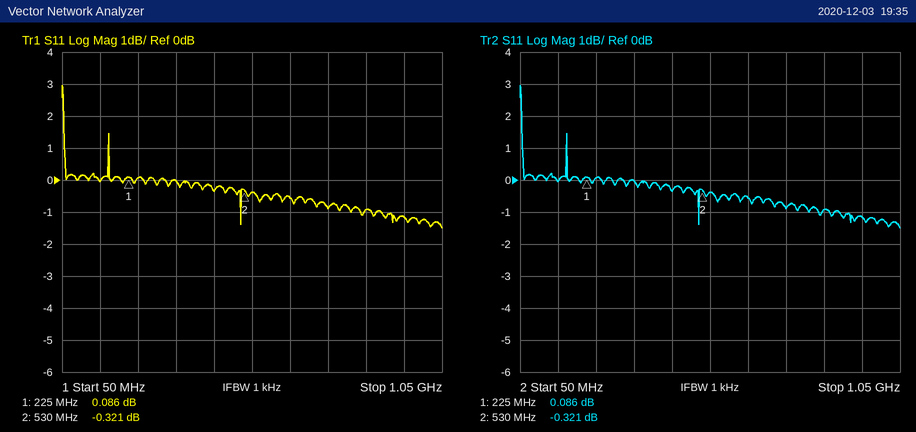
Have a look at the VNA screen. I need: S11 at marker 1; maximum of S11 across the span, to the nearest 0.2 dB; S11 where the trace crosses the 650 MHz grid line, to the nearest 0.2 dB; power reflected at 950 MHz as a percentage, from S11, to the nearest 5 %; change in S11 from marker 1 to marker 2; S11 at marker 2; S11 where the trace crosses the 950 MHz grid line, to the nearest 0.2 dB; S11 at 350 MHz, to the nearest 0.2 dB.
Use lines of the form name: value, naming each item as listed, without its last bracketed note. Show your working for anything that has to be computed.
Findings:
S11 at marker 1: 0.086 dB
maximum of S11 across the span, to the nearest 0.2 dB: 3.0 dB
S11 where the trace crosses the 650 MHz grid line, to the nearest 0.2 dB: -0.6 dB
power reflected at 950 MHz as a percentage, from S11, to the nearest 5 %: 10^(-1.2/10) ≈ 75.9 %, so 75 % to the nearest 5 %
change in S11 from marker 1 to marker 2: -0.321 − (0.086) = -0.407 dB
S11 at marker 2: -0.321 dB
S11 where the trace crosses the 950 MHz grid line, to the nearest 0.2 dB: -1.2 dB
S11 at 350 MHz, to the nearest 0.2 dB: 0.0 dB
